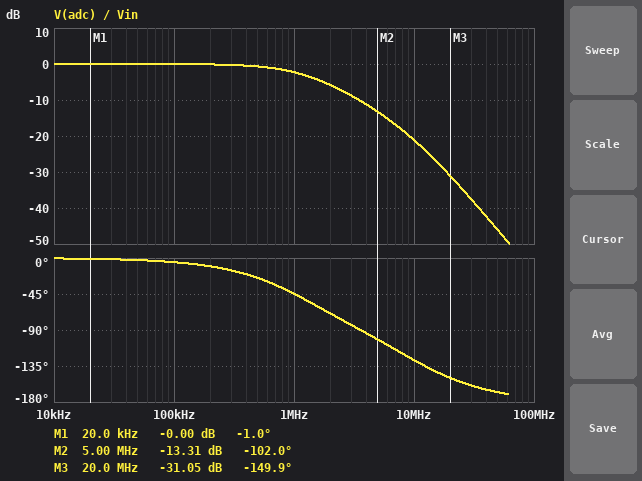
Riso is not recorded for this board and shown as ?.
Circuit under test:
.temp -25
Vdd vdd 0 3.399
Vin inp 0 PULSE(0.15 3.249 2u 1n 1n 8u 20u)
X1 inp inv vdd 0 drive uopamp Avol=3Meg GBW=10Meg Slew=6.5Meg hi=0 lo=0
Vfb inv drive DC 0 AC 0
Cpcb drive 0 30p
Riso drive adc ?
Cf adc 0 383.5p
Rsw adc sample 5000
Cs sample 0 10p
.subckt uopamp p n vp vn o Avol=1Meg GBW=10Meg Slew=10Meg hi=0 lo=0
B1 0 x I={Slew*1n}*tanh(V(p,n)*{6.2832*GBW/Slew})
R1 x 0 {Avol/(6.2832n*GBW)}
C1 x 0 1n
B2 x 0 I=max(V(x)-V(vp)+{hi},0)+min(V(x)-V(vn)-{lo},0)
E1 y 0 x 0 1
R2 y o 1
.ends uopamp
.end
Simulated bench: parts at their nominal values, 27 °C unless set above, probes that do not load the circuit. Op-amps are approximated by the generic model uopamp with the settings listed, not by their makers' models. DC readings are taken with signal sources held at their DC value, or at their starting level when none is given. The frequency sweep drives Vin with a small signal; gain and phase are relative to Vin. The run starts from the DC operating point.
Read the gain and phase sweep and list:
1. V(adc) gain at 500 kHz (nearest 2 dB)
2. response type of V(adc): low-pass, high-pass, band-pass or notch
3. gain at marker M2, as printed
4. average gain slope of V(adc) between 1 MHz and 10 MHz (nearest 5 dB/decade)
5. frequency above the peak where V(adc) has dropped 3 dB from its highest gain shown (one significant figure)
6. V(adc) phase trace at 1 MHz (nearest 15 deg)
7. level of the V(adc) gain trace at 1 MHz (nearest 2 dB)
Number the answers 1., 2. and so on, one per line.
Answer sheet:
1. 0 dB
2. low-pass
3. -13.31 dB
4. -20 dB/decade
5. 1 MHz
6. -45 deg
7. -2 dB
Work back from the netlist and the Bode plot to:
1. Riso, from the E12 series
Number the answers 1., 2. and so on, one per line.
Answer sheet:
1. 330 Ω
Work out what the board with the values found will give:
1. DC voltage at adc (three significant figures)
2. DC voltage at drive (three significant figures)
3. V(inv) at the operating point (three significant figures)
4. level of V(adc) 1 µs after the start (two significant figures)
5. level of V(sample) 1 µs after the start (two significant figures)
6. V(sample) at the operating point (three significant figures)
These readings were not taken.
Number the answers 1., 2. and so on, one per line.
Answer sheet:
1. 150 mV
2. 150 mV
3. 150 mV
4. 150 mV
5. 150 mV
6. 150 mV
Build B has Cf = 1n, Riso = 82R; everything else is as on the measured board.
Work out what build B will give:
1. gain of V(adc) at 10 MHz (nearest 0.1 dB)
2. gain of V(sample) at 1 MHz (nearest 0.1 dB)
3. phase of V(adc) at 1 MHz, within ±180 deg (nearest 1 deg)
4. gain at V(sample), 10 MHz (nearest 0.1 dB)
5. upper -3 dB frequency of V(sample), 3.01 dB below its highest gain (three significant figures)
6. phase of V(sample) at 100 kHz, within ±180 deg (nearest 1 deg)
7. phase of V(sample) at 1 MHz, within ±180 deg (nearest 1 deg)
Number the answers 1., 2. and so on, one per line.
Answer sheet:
1. -17.5 dB
2. -1.5 dB
3. -33 deg
4. -27.8 dB
5. 1.49 MHz
6. -5 deg
7. -51 deg
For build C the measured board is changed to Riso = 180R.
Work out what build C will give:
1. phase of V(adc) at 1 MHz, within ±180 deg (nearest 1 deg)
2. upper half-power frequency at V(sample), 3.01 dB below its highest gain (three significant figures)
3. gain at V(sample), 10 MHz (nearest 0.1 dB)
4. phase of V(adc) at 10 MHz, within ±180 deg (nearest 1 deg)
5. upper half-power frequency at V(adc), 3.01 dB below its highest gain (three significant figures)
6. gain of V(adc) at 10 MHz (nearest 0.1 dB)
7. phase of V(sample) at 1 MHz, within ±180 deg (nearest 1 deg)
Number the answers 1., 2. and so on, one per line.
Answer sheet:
1. -30 deg
2. 1.64 MHz
3. -26.4 dB
4. -122 deg
5. 2.14 MHz
6. -16.0 dB
7. -47 deg
